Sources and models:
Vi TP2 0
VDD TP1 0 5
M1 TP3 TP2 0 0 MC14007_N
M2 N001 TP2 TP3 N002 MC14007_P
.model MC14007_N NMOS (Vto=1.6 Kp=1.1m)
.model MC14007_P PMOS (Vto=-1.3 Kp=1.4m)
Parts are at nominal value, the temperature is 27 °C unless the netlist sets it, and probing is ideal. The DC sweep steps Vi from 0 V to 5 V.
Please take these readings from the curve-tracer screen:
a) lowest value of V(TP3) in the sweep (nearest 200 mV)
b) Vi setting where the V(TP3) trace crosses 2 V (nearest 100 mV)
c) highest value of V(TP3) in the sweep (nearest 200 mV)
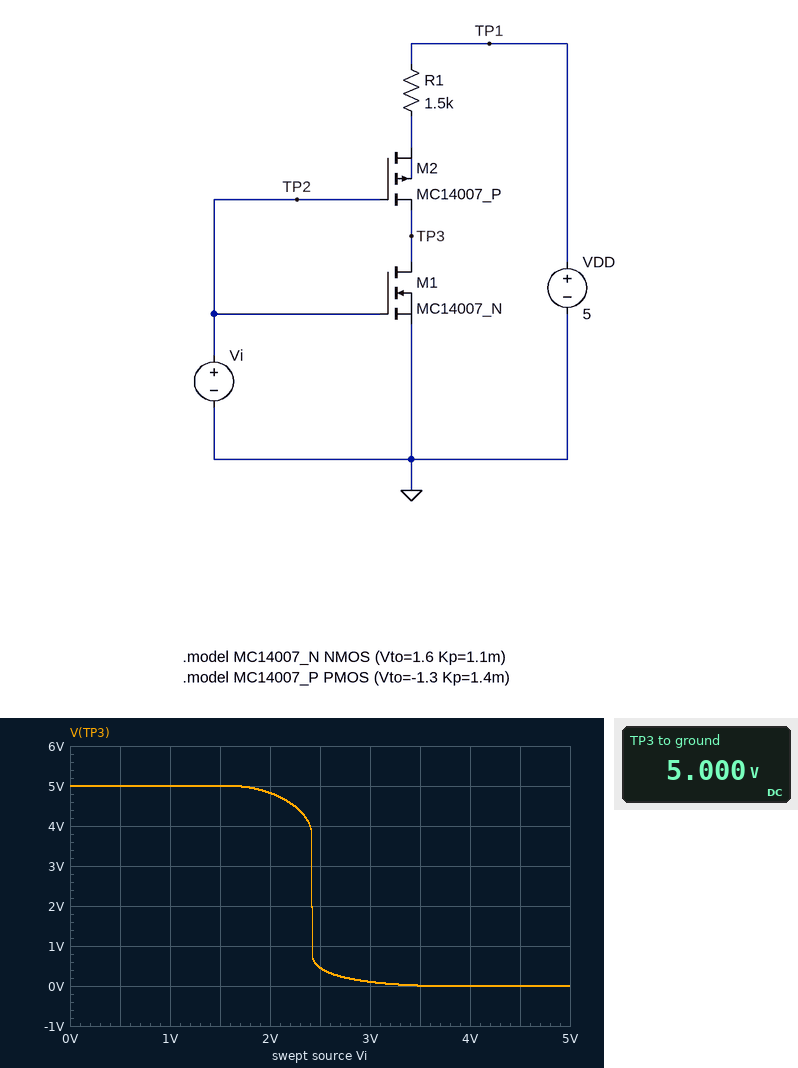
0 V
2.4 V
5.0 V
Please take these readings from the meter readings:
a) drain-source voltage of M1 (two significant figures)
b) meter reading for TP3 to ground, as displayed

5.0 V
5.000 V
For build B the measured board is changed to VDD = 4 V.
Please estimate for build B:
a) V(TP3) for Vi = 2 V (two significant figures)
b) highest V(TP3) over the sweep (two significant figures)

3.7 V
4.0 V
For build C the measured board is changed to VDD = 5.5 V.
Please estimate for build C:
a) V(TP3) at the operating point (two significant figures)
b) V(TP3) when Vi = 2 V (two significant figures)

5.5 V
5.3 V
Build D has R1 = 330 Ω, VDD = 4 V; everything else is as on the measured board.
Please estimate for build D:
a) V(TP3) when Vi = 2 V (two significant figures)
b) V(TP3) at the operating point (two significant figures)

3.9 V
4.0 V
